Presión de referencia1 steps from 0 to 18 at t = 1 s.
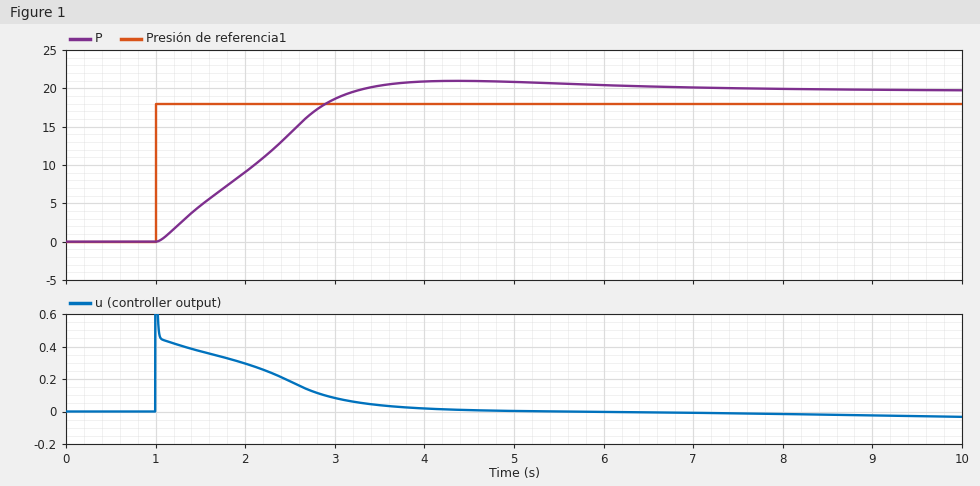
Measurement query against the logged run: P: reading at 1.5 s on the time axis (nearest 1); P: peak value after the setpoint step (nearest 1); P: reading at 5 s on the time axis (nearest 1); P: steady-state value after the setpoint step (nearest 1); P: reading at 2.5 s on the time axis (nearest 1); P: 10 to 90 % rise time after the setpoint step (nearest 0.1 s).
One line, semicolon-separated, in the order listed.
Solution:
5; 21; 21; 20; 14; 1.6 s
